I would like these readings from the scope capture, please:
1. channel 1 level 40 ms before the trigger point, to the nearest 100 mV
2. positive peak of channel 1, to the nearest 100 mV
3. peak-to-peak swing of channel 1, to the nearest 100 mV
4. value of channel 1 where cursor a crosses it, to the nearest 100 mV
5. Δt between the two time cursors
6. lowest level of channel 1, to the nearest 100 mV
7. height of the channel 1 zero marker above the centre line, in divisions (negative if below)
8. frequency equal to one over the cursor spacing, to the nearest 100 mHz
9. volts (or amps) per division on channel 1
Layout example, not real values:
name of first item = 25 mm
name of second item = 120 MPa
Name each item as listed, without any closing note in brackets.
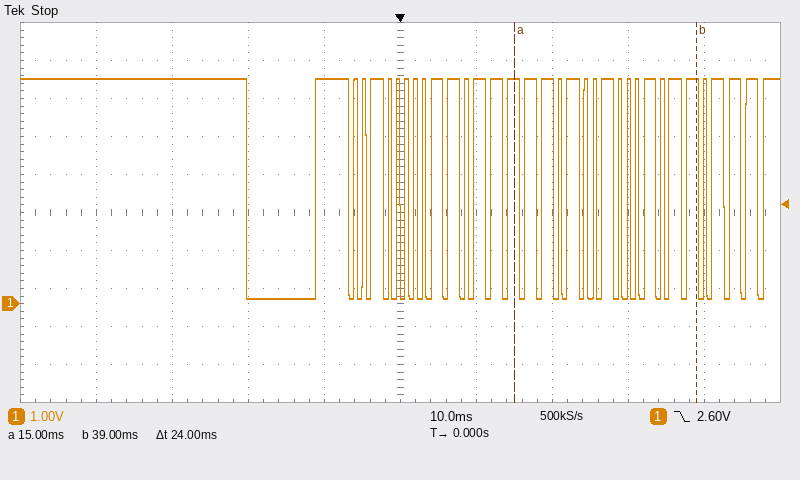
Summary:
channel 1 level 40 ms before the trigger point, to the nearest 100 mV = 5.9 V
positive peak of channel 1, to the nearest 100 mV = 5.9 V
peak-to-peak swing of channel 1, to the nearest 100 mV = 5.8 V
value of channel 1 where cursor a crosses it, to the nearest 100 mV = 5.9 V
Δt between the two time cursors = 24 ms
lowest level of channel 1, to the nearest 100 mV = 100 mV
height of the channel 1 zero marker above the centre line, in divisions = -2.4 div
frequency equal to one over the cursor spacing, to the nearest 100 mHz = 41.7 Hz
volts (or amps) per division on channel 1 = 1 V
